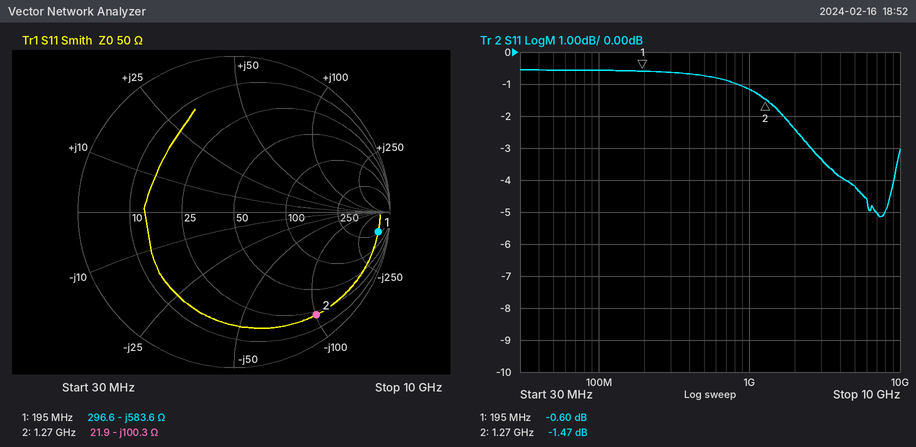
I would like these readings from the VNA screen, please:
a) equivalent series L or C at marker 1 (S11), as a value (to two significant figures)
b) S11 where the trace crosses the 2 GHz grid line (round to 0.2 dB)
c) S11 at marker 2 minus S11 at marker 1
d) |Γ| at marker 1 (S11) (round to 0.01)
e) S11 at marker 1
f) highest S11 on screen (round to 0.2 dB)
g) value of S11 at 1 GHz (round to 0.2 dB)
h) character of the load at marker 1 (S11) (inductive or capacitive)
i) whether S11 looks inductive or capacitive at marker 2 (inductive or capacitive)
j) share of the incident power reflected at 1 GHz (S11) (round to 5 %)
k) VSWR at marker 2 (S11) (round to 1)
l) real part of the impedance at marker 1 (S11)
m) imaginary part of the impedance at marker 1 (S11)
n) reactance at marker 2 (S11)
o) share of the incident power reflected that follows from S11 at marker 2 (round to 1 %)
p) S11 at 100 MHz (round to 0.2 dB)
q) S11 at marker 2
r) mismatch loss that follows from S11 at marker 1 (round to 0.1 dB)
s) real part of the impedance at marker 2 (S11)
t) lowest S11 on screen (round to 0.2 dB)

1.4 pF
-2.4 dB
-0.87 dB
0.93
-0.60 dB
-0.6 dB
-1.2 dB
capacitive
capacitive
75 %
12
296.6 Ω
-583.6 Ω
-100.3 Ω
71 %
-0.6 dB
-1.47 dB
8.9 dB
21.9 Ω
-5.2 dB
